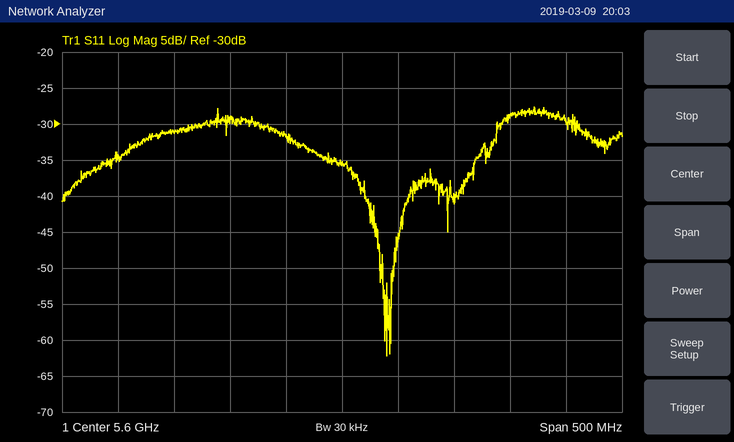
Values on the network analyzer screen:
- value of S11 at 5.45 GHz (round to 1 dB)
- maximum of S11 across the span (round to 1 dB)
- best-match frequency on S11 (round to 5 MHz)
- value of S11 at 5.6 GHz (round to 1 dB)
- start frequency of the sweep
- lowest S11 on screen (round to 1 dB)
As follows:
-31 dB
-28 dB
5.640 GHz
-35 dB
5.35 GHz
-62 dB
